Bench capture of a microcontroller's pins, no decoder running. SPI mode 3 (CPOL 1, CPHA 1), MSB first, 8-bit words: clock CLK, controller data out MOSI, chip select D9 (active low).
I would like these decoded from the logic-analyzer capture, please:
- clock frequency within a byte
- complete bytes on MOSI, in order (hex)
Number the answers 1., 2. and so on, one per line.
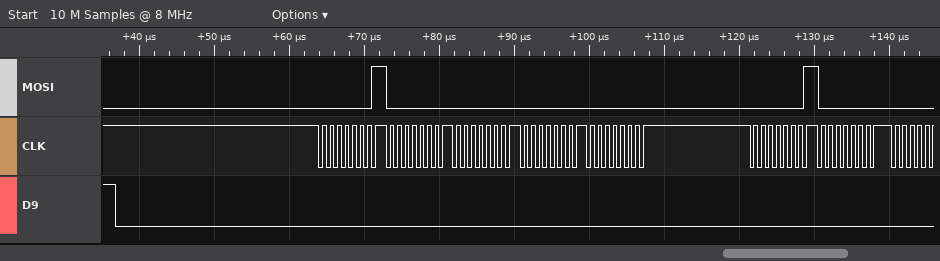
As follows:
1. 1 MHz
2. 0x01 0x00 0x00 0x00 0x00 0x01 0x00
